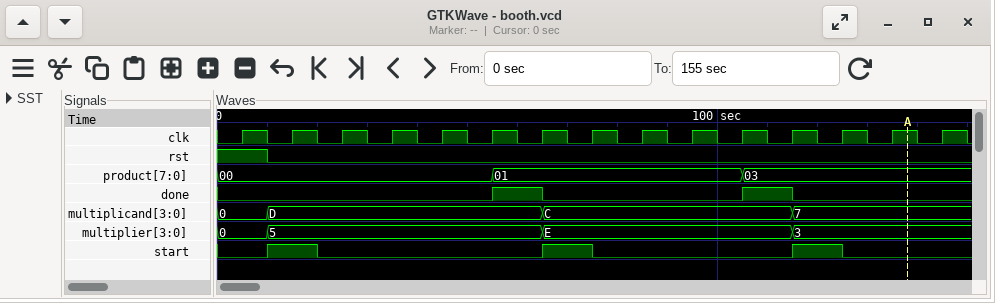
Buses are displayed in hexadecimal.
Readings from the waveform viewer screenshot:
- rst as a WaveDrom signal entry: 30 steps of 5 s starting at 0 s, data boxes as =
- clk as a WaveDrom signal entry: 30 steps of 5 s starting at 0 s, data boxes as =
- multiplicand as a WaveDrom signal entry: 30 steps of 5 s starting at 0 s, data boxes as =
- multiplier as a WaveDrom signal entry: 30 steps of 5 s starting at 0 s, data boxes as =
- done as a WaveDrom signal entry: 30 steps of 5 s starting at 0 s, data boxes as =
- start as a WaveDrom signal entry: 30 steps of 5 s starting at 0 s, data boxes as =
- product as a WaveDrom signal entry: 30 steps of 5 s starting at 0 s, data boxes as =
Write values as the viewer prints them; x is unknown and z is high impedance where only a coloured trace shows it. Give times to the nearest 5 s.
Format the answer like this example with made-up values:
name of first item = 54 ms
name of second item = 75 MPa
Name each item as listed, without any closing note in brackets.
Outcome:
rst as a WaveDrom signal entry: 30 steps of 5 s starting at 0 s, data boxes as = = {name: 'rst', wave: '1.0...........................'}
clk as a WaveDrom signal entry: 30 steps of 5 s starting at 0 s, data boxes as = = {name: 'clk', wave: '010101010101010101010101010101'}
multiplicand as a WaveDrom signal entry: 30 steps of 5 s starting at 0 s, data boxes as = = {name: 'multiplicand', wave: '=.=..........=.........=......', data: '0 D C 7'}
multiplier as a WaveDrom signal entry: 30 steps of 5 s starting at 0 s, data boxes as = = {name: 'multiplier', wave: '=.=..........=.........=......', data: '0 5 E 3'}
done as a WaveDrom signal entry: 30 steps of 5 s starting at 0 s, data boxes as = = {name: 'done', wave: '0..........1.0.......1.0......'}
start as a WaveDrom signal entry: 30 steps of 5 s starting at 0 s, data boxes as = = {name: 'start', wave: '0.1.0........1.0.......1.0....'}
product as a WaveDrom signal entry: 30 steps of 5 s starting at 0 s, data boxes as = = {name: 'product', wave: '=..........=.........=........', data: '00 01 03'}
